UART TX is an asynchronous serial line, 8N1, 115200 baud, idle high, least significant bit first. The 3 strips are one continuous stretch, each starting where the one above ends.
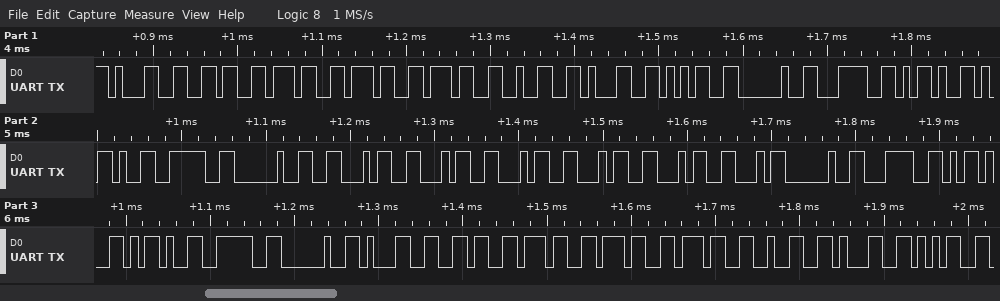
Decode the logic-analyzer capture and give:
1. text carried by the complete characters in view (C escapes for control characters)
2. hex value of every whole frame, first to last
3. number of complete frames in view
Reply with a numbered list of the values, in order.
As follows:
1. "16777215 <--> FFFFFF <--> 16777215"
2. 31 36 37 37 37 32 31 35 20 3C 2D 2D 3E 20 46 46 46 46 46 46 20 3C 2D 2D 3E 20 31 36 37 37 37 32 31 35
3. 34
